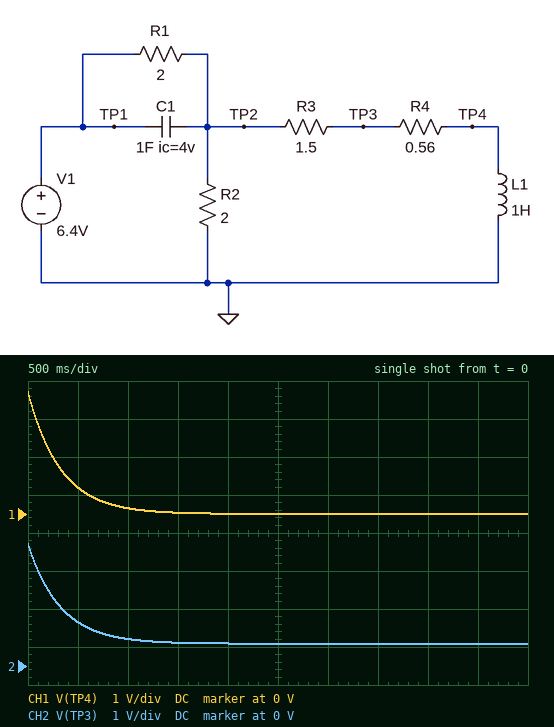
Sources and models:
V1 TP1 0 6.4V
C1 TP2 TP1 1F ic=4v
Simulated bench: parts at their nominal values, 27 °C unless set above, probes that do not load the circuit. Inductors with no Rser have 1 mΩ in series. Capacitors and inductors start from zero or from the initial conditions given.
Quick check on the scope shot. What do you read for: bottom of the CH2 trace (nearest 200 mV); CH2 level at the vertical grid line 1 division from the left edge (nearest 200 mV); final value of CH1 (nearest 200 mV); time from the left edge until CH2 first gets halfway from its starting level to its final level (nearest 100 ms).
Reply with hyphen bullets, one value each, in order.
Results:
- 600 mV
- 1.2 V
- 0 V
- 200 ms
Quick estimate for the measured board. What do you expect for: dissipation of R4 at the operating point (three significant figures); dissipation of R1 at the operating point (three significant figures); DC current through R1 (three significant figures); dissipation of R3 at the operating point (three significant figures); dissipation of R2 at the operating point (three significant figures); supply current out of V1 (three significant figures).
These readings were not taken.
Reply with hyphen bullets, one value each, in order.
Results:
- 612 mW
- 9.01 W
- 2.12 A
- 1.64 W
- 2.32 W
- 2.12 A
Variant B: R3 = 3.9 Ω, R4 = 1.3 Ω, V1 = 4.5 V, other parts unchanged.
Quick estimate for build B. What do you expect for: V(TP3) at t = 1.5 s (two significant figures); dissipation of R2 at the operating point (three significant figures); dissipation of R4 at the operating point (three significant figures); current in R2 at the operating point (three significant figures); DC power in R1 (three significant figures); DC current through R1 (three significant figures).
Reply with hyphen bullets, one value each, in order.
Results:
- 470 mV
- 1.78 W
- 171 mW
- 944 mA
- 3.41 W
- 1.31 A
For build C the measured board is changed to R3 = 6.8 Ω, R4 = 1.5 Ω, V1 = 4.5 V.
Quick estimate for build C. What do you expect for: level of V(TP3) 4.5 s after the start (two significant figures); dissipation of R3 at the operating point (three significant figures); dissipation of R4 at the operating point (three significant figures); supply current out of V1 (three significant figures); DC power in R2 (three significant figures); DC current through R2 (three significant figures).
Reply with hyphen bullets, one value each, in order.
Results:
- 360 mV
- 398 mW
- 87.8 mW
- 1.25 A
- 2.02 W
- 1.00 A
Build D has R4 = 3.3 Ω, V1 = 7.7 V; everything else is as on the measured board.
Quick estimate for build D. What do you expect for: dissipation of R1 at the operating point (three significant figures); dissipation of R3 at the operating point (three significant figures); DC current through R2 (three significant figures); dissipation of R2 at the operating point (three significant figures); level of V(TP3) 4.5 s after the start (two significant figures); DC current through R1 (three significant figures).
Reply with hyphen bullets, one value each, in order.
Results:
- 10.2 W
- 661 mW
- 1.59 A
- 5.08 W
- 2.2 V
- 2.26 A
